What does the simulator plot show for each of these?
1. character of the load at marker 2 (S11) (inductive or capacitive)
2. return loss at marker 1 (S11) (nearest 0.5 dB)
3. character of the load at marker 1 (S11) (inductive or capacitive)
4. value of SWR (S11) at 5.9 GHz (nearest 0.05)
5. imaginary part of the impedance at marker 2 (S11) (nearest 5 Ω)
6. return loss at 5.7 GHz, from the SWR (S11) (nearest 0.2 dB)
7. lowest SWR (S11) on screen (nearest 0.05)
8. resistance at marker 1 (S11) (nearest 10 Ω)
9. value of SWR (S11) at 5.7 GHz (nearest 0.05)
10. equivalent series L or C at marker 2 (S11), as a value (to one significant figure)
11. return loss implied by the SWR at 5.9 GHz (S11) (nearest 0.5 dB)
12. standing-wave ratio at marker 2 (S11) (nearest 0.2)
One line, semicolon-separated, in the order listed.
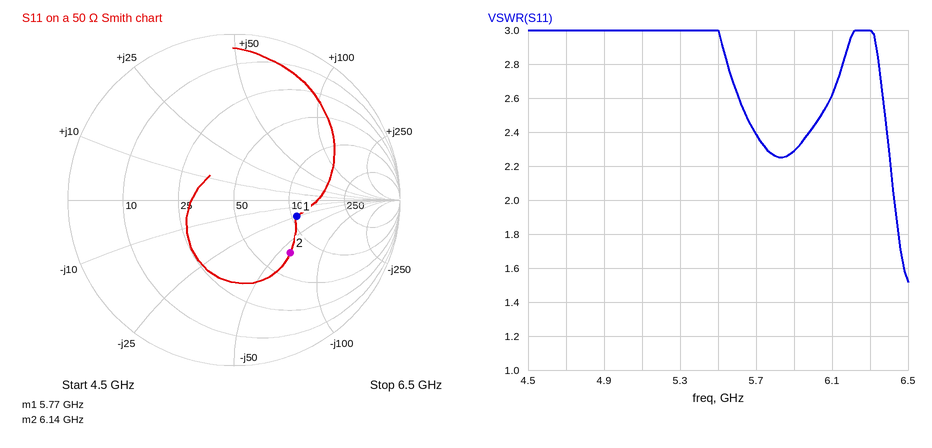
capacitive; 8.0 dB; capacitive; 2.30; -60 Ω; 7.8 dB; 1.50; 110 Ω; 2.40; 400 fF; 8.0 dB; 2.8
